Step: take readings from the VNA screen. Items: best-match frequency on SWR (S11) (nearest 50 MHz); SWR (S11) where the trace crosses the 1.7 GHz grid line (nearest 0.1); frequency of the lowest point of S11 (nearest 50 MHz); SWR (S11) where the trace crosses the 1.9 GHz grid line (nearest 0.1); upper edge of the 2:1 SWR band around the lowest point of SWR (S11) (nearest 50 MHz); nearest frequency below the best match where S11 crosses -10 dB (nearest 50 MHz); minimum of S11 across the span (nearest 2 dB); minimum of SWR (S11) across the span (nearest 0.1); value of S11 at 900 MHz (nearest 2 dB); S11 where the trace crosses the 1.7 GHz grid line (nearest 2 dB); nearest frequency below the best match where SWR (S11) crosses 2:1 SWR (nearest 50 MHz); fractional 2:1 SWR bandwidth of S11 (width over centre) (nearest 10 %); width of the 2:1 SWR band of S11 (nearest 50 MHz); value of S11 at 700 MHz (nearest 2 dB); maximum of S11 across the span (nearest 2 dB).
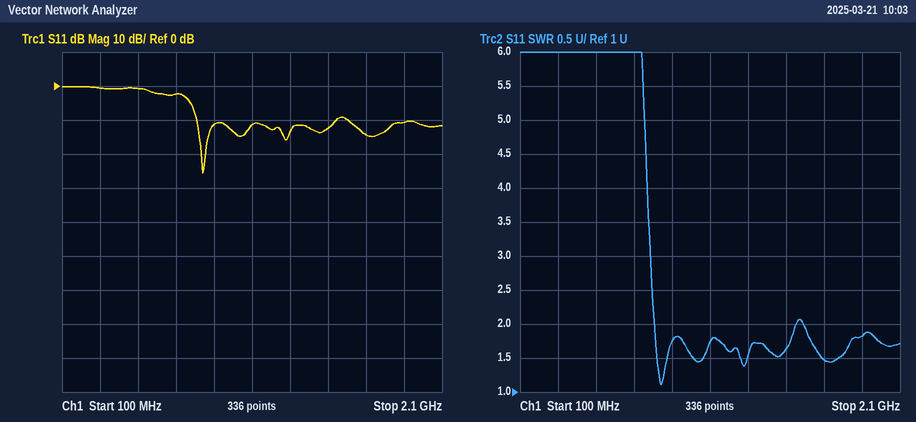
850 MHz
1.5
850 MHz
1.8
1.55 GHz
800 MHz
-26 dB
1.1
-12 dB
-14 dB
800 MHz
60 %
750 MHz
-2 dB
0 dB
